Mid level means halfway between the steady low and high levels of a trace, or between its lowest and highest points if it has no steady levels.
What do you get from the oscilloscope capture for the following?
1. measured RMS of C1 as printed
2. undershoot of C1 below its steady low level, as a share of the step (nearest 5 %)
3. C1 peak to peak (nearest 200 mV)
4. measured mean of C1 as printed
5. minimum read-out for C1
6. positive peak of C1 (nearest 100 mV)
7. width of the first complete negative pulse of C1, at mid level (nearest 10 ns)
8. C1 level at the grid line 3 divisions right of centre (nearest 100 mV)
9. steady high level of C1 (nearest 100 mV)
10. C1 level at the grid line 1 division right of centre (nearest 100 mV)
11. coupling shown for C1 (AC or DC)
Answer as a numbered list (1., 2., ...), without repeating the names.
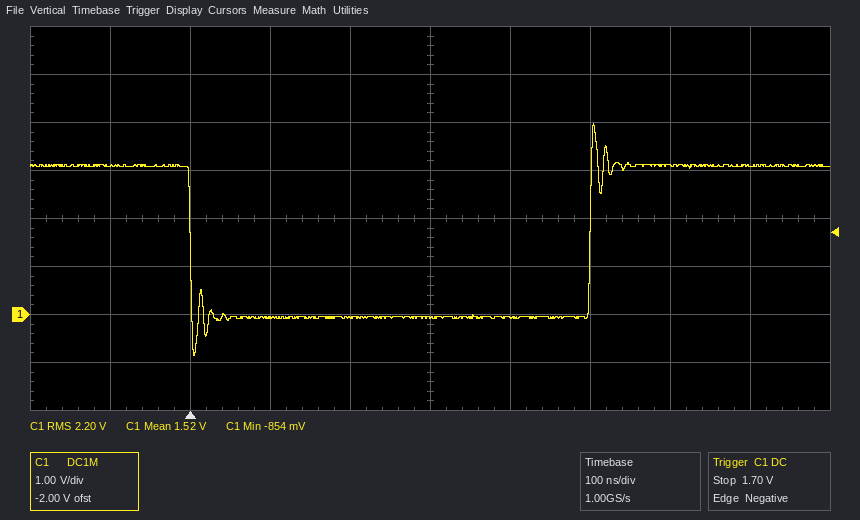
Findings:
1. 2.20 V
2. 25 %
3. 4.8 V
4. 1.52 V
5. -854 mV
6. 4.0 V
7. 500 ns
8. 3.1 V
9. 3.1 V
10. -100 mV
11. DC
